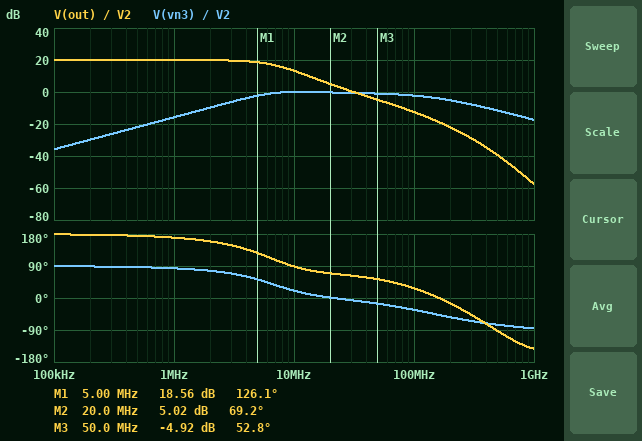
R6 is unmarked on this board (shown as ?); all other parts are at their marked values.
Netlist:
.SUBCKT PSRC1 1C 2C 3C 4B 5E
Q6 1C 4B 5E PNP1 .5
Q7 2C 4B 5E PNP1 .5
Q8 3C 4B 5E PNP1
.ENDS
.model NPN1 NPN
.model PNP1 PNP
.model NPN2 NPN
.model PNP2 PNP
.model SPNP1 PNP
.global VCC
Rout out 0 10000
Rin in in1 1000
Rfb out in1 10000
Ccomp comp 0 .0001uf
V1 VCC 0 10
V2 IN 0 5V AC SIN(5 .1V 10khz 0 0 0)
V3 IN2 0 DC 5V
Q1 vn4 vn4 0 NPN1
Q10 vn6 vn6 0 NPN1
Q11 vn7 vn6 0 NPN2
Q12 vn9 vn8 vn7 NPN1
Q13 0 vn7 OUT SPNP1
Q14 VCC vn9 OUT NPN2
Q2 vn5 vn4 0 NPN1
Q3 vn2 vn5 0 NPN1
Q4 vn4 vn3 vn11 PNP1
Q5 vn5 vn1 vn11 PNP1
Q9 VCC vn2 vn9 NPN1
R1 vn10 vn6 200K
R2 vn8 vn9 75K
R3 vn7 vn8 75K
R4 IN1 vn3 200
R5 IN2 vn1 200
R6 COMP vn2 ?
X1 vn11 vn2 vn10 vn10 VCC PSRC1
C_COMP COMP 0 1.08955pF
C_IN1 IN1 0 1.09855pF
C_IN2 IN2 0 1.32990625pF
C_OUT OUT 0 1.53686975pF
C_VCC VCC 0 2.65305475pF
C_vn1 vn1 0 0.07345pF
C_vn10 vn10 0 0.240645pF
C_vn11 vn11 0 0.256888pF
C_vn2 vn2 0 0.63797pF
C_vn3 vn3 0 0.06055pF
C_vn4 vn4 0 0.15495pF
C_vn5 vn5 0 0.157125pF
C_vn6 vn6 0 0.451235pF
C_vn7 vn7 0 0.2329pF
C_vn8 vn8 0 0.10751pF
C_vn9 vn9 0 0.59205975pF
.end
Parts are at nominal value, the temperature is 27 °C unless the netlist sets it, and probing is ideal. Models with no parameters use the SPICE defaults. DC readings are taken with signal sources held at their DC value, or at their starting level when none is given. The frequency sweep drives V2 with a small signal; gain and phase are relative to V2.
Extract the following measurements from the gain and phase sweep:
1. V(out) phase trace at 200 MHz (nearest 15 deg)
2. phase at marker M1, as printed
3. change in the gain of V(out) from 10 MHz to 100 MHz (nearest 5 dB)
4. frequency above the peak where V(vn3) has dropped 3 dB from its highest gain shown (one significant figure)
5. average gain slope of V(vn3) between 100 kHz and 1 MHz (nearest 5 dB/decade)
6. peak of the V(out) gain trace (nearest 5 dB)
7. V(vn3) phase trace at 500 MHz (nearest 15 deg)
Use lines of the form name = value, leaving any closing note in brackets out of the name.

V(out) phase trace at 200 MHz = -15 deg
phase at marker M1, as printed = 126.1 deg
change in the gain of V(out) from 10 MHz to 100 MHz = -25 dB
frequency above the peak where V(vn3) has dropped 3 dB from its highest gain shown = 100 MHz
average gain slope of V(vn3) between 100 kHz and 1 MHz = 20 dB/decade
peak of the V(out) gain trace = 20 dB
V(vn3) phase trace at 500 MHz = -75 deg
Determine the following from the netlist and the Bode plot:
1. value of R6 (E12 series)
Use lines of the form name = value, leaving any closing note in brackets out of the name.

value of R6 = 100 Ω
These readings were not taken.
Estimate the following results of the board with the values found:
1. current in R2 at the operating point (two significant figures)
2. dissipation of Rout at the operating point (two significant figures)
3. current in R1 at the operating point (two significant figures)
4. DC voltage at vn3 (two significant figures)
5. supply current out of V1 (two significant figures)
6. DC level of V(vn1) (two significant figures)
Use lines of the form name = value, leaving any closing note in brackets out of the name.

current in R2 at the operating point = 9.5 µA
dissipation of Rout at the operating point = 2.5 mW
current in R1 at the operating point = 43 µA
DC voltage at vn3 = 5.0 V
supply current out of V1 = 630 µA
DC level of V(vn1) = 5.0 V
